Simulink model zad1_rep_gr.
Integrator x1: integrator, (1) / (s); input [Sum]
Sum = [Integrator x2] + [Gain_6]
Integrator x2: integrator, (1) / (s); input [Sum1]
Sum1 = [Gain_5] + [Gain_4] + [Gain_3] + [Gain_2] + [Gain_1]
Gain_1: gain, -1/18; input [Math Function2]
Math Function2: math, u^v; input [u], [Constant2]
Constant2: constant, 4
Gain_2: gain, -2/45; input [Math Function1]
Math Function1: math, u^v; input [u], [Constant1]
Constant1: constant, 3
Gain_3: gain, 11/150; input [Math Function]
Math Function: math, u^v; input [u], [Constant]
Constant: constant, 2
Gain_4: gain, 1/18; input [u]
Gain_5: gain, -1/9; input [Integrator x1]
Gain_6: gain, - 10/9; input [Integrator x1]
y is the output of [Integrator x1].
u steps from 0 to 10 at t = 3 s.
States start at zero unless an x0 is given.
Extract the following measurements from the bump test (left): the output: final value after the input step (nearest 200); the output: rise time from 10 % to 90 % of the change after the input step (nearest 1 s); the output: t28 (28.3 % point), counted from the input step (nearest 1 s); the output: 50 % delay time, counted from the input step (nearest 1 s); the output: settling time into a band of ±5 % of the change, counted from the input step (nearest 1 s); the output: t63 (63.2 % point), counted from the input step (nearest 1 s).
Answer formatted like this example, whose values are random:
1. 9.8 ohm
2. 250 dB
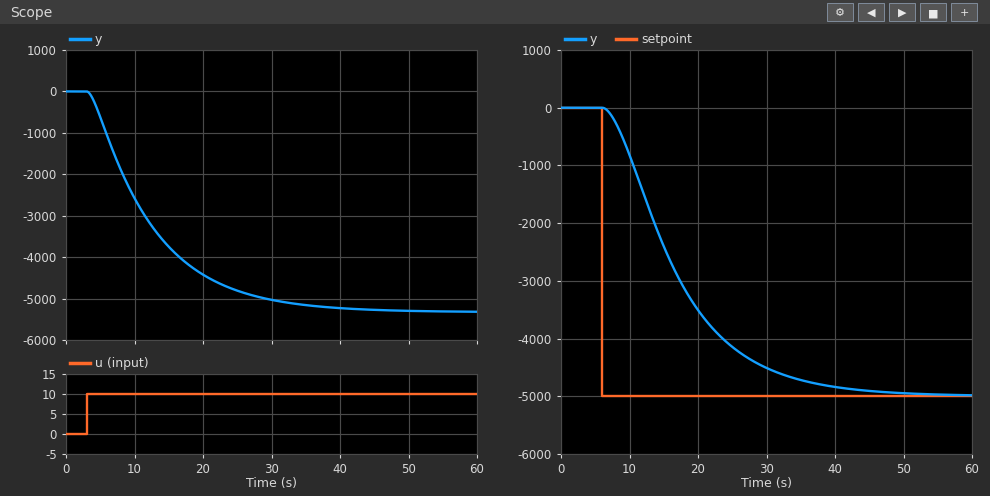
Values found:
1. -5400
2. 20 s
3. 4 s
4. 7 s
5. 28 s
6. 10 s
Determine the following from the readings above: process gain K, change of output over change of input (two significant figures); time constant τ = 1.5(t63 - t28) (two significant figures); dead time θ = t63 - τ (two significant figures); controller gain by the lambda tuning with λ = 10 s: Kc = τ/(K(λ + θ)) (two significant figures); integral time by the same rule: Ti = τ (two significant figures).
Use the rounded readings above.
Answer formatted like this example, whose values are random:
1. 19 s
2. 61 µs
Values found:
1. -540
2. 9.0 s
3. 1.0 s
4. -0.0015
5. 9.0 s
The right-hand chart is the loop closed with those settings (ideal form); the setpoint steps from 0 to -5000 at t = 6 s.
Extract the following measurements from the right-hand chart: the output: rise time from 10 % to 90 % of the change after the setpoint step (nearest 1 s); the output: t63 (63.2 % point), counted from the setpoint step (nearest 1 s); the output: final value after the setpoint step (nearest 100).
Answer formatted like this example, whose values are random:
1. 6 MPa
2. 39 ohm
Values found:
1. 21 s
2. 12 s
3. -5000
